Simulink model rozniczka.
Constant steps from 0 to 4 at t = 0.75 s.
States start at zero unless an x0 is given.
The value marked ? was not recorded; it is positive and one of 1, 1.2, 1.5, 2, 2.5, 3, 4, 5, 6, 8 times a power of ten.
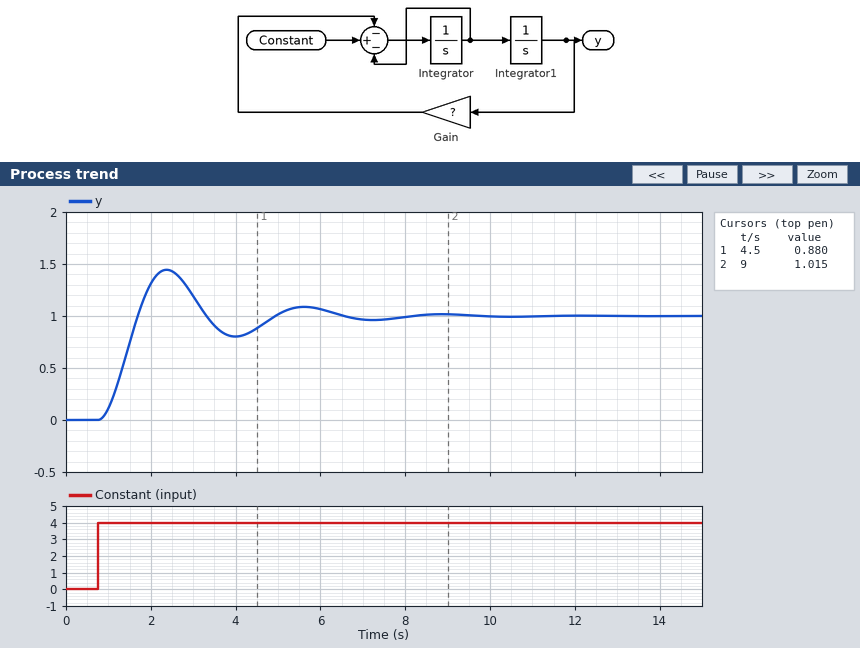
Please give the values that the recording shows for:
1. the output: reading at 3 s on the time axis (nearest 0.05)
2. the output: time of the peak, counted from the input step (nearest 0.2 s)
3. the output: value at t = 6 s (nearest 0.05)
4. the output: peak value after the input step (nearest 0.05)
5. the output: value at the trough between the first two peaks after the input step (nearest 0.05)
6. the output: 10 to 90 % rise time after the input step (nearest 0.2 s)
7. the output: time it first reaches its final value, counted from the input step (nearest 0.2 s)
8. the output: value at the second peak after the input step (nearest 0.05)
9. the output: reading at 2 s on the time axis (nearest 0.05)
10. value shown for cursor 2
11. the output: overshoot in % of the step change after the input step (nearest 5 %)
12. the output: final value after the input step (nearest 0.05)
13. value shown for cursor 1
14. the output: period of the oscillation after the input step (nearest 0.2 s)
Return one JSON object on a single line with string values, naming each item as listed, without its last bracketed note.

{"the output: reading at 3 s on the time axis": "1.20", "the output: time of the peak, counted from the input step": "1.6 s", "the output: value at t = 6 s": "1.05", "the output: peak value after the input step": "1.45", "the output: value at the trough between the first two peaks after the input step": "0.80", "the output: 10 to 90 % rise time after the input step": "0.6 s", "the output: time it first reaches its final value, counted from the input step": "1.0 s", "the output: value at the second peak after the input step": "1.10", "the output: reading at 2 s on the time axis": "1.30", "value shown for cursor 2": "1.015", "the output: overshoot in % of the step change after the input step": "45 %", "the output: final value after the input step": "1.00", "value shown for cursor 1": "0.880", "the output: period of the oscillation after the input step": "3.2 s"}
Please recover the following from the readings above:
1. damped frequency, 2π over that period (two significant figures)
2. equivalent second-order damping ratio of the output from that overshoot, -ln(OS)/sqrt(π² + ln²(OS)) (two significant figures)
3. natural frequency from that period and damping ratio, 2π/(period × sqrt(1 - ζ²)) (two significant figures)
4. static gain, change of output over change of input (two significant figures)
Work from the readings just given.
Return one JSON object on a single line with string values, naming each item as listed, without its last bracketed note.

{"damped frequency, 2π over that period": "2.0 rad/s", "equivalent second-order damping ratio of the output from that overshoot, -ln(OS)/sqrt(π² + ln²(OS))": "0.25", "natural frequency from that period and damping ratio, 2π/(period × sqrt(1 - ζ²))": "2.0 rad/s", "static gain, change of output over change of input": "0.25"}
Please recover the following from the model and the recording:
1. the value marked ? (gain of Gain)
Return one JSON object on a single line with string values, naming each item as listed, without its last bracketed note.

{"the value marked ?": "4"}
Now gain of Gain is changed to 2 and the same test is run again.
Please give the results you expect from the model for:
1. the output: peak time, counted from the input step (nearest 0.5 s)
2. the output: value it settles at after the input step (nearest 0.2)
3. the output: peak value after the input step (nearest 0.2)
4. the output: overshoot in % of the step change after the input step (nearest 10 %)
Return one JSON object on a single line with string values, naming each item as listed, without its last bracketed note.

{"the output: peak time, counted from the input step": "2.5 s", "the output: value it settles at after the input step": "2.0", "the output: peak value after the input step": "2.6", "the output: overshoot in % of the step change after the input step": "30 %"}
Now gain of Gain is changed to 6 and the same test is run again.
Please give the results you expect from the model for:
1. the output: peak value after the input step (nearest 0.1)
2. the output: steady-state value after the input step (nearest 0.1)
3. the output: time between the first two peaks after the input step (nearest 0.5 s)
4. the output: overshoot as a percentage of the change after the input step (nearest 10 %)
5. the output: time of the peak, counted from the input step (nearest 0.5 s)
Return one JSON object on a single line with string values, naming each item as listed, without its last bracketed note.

{"the output: peak value after the input step": "1.0", "the output: steady-state value after the input step": "0.7", "the output: time between the first two peaks after the input step": "2.5 s", "the output: overshoot as a percentage of the change after the input step": "50 %", "the output: time of the peak, counted from the input step": "1.5 s"}
